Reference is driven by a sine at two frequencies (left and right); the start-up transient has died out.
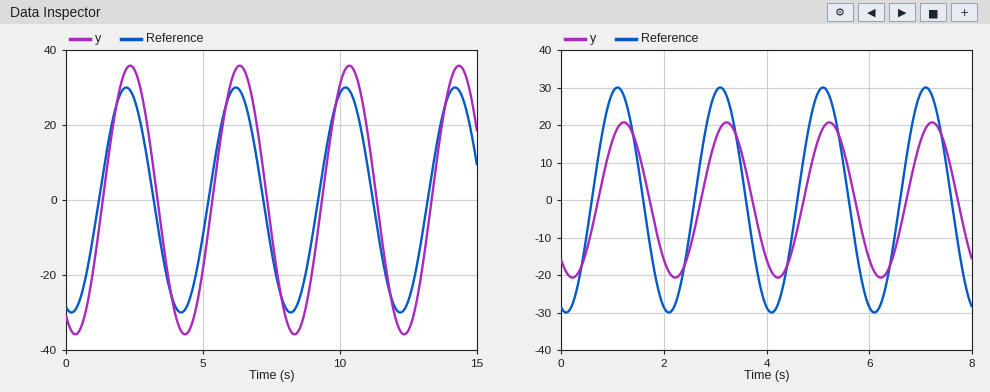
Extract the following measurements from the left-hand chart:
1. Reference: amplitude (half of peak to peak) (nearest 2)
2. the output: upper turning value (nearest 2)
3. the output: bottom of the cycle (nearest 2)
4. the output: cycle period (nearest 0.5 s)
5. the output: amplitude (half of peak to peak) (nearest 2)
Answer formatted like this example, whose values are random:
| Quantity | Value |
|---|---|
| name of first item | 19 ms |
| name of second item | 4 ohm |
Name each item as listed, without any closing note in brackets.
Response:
| Quantity | Value |
|---|---|
| Reference: amplitude (half of peak to peak) | 30 |
| the output: upper turning value | 36 |
| the output: bottom of the cycle | -36 |
| the output: cycle period | 4.0 s |
| the output: amplitude (half of peak to peak) | 36 |
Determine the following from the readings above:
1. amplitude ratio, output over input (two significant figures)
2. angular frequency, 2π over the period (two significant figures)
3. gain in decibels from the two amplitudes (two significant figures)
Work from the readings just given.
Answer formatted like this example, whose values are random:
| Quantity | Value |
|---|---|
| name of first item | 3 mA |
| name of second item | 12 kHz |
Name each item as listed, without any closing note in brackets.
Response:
| Quantity | Value |
|---|---|
| amplitude ratio, output over input | 1.2 |
| angular frequency, 2π over the period | 1.6 rad/s |
| gain in decibels from the two amplitudes | 1.6 dB |
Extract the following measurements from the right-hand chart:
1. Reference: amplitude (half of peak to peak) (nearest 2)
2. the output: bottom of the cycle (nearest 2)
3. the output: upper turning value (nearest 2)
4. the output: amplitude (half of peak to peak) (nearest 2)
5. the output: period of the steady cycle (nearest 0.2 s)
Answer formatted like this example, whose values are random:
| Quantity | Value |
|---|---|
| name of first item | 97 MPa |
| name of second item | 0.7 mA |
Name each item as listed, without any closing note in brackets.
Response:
| Quantity | Value |
|---|---|
| Reference: amplitude (half of peak to peak) | 30 |
| the output: bottom of the cycle | -20 |
| the output: upper turning value | 20 |
| the output: amplitude (half of peak to peak) | 20 |
| the output: period of the steady cycle | 2.0 s |
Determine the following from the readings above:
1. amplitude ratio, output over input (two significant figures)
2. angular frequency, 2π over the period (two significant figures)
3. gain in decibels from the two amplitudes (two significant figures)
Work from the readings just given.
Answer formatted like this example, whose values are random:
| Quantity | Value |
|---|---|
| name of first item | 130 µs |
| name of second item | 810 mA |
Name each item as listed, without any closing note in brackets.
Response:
| Quantity | Value |
|---|---|
| amplitude ratio, output over input | 0.67 |
| angular frequency, 2π over the period | 3.1 rad/s |
| gain in decibels from the two amplitudes | -3.5 dB |
